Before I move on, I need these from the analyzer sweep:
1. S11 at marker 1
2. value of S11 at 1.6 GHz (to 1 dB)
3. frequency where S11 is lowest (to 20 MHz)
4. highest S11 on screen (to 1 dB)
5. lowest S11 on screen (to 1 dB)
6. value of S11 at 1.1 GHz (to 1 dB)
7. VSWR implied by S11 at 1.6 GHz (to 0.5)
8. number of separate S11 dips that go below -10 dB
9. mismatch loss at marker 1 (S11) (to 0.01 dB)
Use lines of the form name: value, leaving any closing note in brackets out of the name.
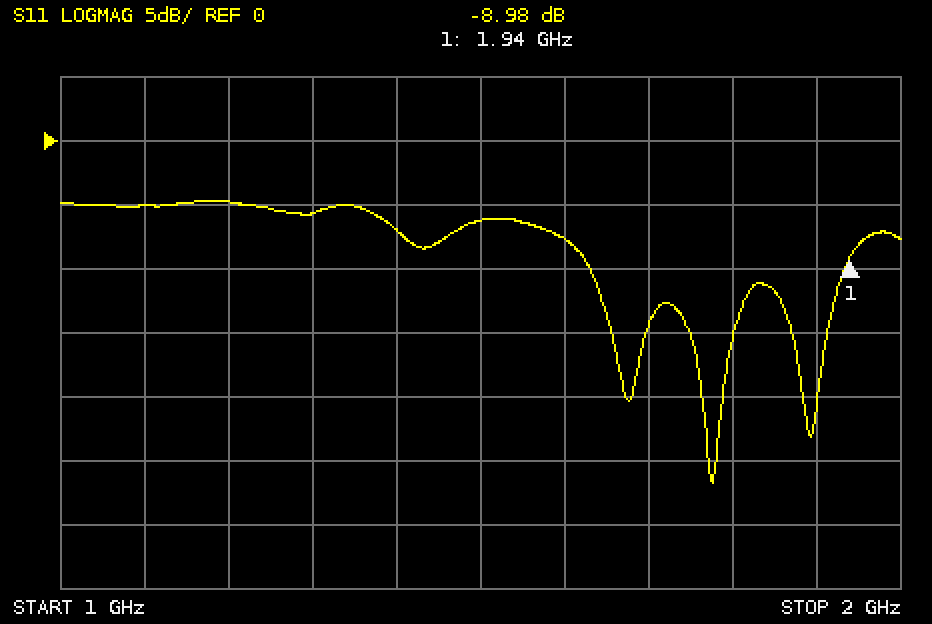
S11 at marker 1: -8.98 dB
value of S11 at 1.6 GHz: -8 dB
frequency where S11 is lowest: 1.78 GHz
highest S11 on screen: -5 dB
lowest S11 on screen: -27 dB
value of S11 at 1.1 GHz: -5 dB
VSWR implied by S11 at 1.6 GHz: 2.5
number of separate S11 dips that go below -10 dB: 3
mismatch loss at marker 1 (S11): 0.59 dB
